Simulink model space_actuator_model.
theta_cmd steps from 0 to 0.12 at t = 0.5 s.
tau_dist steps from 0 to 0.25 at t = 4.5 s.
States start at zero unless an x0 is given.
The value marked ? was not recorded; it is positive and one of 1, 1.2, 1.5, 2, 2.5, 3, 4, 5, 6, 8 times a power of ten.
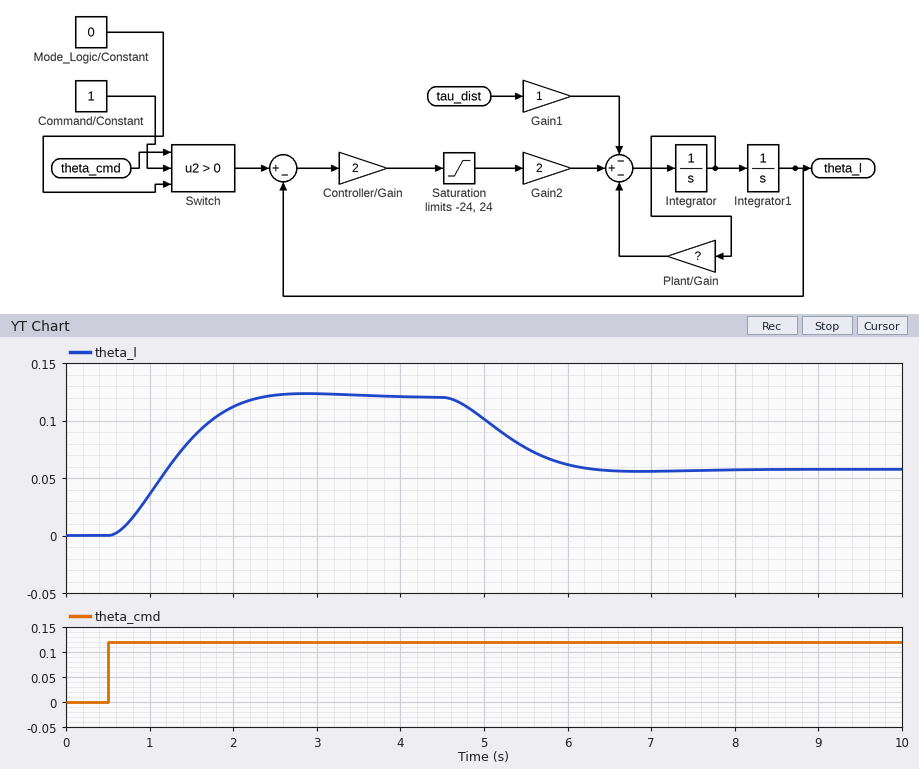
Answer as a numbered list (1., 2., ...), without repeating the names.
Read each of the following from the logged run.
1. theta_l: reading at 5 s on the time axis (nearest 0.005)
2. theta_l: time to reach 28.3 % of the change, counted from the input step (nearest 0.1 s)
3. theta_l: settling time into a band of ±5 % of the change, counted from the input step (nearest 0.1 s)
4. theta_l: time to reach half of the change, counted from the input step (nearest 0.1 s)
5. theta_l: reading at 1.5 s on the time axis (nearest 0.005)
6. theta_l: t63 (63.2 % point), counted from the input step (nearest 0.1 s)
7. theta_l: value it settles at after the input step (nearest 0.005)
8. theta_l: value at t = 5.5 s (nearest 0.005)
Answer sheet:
1. 0.100
2. 0.5 s
3. 1.6 s
4. 0.7 s
5. 0.085
6. 0.9 s
7. 0.120
8. 0.075
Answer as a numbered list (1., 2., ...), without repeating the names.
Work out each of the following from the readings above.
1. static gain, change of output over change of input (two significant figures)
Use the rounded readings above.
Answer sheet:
1. 1.0
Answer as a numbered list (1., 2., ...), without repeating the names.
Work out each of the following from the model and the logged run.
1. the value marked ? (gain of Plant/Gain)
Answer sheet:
1. 3
